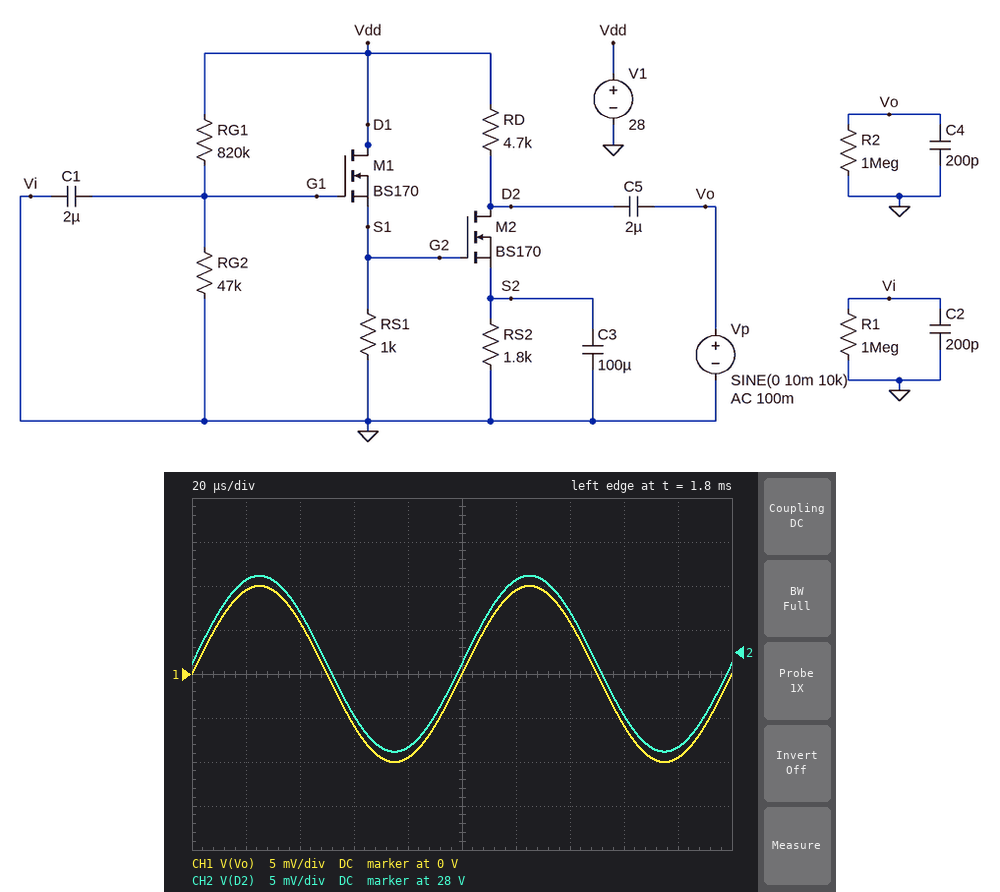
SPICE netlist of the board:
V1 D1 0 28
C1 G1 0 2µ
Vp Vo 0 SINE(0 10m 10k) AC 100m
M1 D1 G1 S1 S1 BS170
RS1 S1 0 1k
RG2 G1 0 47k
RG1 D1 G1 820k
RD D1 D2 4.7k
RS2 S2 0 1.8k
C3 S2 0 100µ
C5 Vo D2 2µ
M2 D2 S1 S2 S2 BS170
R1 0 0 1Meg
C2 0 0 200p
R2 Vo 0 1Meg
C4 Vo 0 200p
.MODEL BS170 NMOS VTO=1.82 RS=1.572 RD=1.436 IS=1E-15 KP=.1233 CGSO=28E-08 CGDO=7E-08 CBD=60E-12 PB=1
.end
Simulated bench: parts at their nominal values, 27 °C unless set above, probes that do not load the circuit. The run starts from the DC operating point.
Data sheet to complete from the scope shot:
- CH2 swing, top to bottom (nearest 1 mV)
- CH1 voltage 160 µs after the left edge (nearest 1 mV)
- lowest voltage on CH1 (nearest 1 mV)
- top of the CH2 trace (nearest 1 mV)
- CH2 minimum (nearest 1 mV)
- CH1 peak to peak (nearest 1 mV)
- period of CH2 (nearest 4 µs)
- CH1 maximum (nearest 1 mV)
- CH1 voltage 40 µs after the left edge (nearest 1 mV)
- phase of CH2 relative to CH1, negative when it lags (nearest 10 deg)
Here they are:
20 mV
-6 mV
-10 mV
28.009 V
27.989 V
20 mV
100 µs
10 mV
6 mV
0 deg
